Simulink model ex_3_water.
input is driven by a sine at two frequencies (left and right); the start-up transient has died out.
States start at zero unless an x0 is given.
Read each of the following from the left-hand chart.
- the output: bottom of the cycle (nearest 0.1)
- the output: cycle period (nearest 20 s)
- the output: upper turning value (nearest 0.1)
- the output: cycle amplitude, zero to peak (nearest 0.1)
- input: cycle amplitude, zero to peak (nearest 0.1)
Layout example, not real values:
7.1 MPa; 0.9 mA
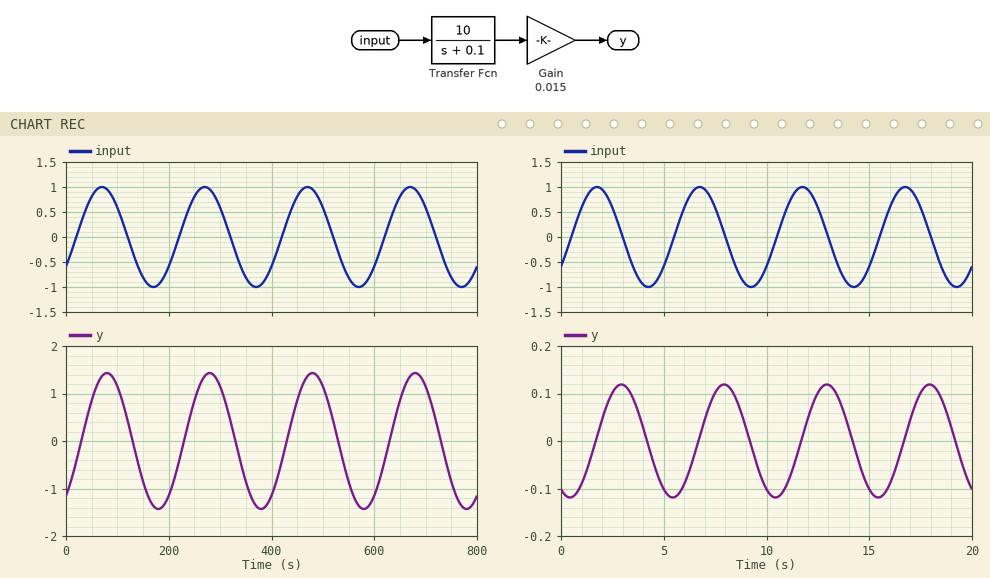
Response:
-1.4; 200 s; 1.4; 1.4; 1.0
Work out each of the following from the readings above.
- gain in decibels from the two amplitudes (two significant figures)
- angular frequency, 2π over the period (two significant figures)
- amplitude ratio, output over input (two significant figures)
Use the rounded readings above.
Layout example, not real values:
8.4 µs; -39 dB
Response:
2.9 dB; 0.031 rad/s; 1.4
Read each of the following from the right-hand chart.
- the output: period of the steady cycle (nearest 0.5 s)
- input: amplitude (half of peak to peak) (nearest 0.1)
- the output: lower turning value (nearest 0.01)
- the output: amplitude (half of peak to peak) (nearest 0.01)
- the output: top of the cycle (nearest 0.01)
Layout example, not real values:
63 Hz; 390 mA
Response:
5.0 s; 1.0; -0.12; 0.12; 0.12
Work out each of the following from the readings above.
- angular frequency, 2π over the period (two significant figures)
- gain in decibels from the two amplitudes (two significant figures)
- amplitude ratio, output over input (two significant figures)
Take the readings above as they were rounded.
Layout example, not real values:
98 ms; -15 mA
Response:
1.3 rad/s; -18 dB; 0.12
